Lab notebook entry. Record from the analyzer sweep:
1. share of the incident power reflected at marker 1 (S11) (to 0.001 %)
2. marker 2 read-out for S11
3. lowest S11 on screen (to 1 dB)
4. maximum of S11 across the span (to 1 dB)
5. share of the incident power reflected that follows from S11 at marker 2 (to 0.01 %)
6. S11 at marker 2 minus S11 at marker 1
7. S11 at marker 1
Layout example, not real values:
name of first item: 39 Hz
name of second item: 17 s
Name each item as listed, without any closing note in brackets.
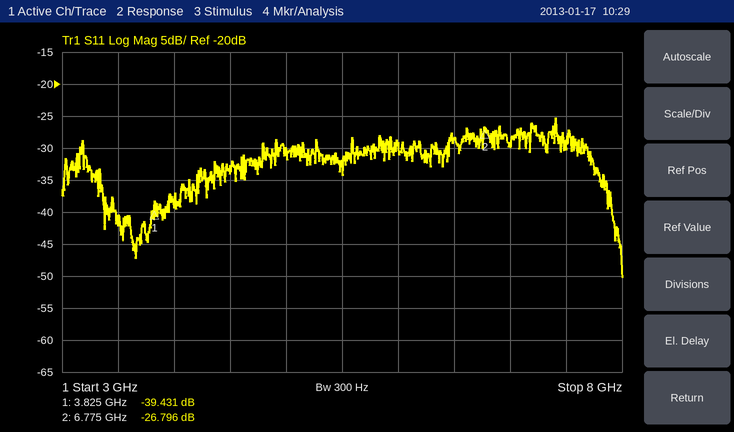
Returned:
share of the incident power reflected at marker 1 (S11): 0.011 %
marker 2 read-out for S11: -26.796 dB
lowest S11 on screen: -50 dB
maximum of S11 across the span: -25 dB
share of the incident power reflected that follows from S11 at marker 2: 0.21 %
S11 at marker 2 minus S11 at marker 1: 12.635 dB
S11 at marker 1: -39.431 dB
